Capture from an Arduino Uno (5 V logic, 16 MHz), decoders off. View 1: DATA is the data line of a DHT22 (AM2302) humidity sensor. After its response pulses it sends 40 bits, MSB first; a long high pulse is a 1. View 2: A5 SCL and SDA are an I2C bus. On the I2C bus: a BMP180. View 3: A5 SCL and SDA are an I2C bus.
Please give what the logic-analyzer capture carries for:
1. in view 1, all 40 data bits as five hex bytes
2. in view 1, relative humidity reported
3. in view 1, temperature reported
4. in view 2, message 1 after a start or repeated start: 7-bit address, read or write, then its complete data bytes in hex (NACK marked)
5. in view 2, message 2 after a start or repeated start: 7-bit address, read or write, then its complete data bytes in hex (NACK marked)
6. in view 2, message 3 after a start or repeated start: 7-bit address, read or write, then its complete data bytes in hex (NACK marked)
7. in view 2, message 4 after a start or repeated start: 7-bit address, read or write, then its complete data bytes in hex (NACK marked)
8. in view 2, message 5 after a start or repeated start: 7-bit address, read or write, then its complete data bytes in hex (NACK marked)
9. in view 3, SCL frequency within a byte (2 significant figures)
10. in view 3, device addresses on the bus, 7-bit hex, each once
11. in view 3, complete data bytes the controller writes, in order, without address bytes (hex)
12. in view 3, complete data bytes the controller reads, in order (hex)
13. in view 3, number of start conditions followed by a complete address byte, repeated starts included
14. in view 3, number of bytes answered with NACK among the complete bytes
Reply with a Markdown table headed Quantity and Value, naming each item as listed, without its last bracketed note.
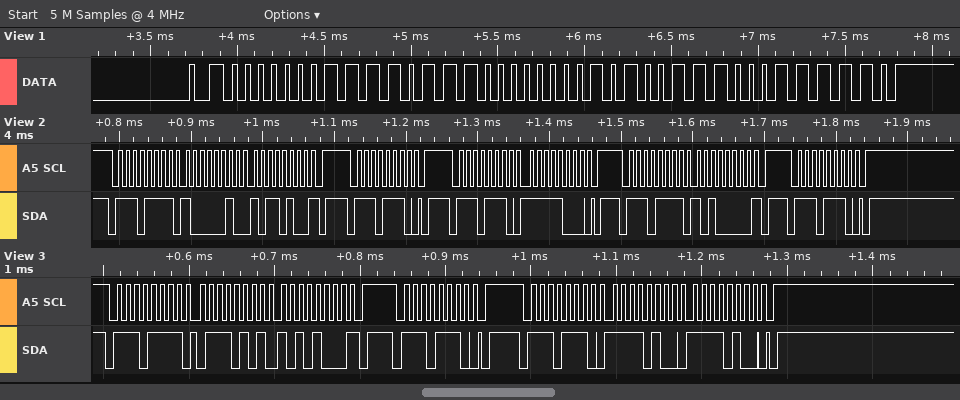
| Quantity | Value |
|---|---|
| in view 1, all 40 data bits as five hex bytes | 01 EE 01 4E 3E |
| in view 1, relative humidity reported | 49.4 % |
| in view 1, temperature reported | 33.4 °C |
| in view 2, message 1 after a start or repeated start: 7-bit address, read or write, then its complete data bytes in hex | 0x77 read: 82 B4 NACK |
| in view 2, message 2 after a start or repeated start: 7-bit address, read or write, then its complete data bytes in hex | 0x77 write |
| in view 2, message 3 after a start or repeated start: 7-bit address, read or write, then its complete data bytes in hex | 0x77 write: F8 |
| in view 2, message 4 after a start or repeated start: 7-bit address, read or write, then its complete data bytes in hex | 0x77 read: A0 NACK |
| in view 2, message 5 after a start or repeated start: 7-bit address, read or write, then its complete data bytes in hex | 0x77 write |
| in view 3, SCL frequency within a byte | 100 kHz |
| in view 3, device addresses on the bus, 7-bit hex, each once | 0x77 |
| in view 3, complete data bytes the controller writes, in order, without address bytes | F4 F4 |
| in view 3, complete data bytes the controller reads, in order | 75 A8 |
| in view 3, number of start conditions followed by a complete address byte, repeated starts included | 3 |
| in view 3, number of bytes answered with NACK among the complete bytes | 1 |
